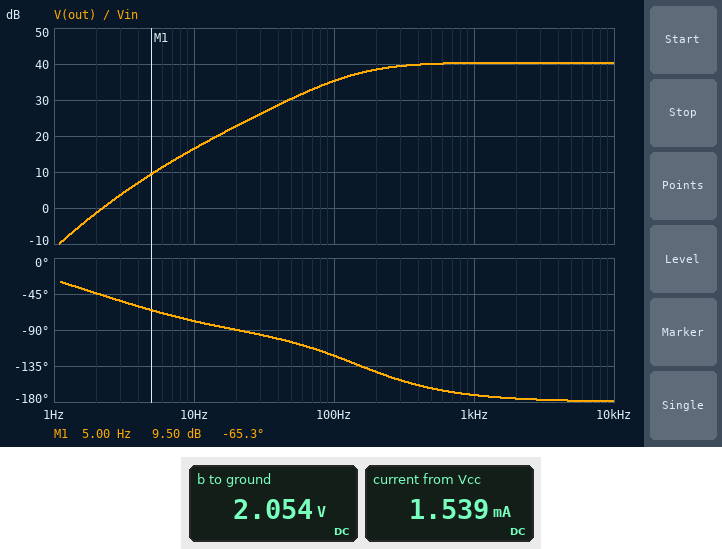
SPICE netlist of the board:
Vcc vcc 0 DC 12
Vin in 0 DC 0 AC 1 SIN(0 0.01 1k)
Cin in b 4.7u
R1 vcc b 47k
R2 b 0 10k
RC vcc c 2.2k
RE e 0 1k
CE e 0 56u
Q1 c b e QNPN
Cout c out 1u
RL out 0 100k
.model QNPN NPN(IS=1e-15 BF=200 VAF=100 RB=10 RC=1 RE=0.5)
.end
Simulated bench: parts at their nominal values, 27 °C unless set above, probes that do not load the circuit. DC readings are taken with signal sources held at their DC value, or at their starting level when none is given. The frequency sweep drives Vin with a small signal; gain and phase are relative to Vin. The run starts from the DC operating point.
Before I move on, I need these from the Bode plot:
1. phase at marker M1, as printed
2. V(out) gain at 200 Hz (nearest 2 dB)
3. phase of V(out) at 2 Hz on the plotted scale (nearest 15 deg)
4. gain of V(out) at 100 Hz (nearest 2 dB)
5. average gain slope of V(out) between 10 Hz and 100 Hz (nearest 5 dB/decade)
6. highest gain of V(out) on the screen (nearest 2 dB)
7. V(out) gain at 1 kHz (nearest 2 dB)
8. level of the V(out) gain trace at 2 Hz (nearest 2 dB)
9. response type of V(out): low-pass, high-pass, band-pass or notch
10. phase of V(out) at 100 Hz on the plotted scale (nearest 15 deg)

-65.3 deg
38 dB
-45 deg
36 dB
20 dB/decade
40 dB
40 dB
-2 dB
high-pass
-120 deg
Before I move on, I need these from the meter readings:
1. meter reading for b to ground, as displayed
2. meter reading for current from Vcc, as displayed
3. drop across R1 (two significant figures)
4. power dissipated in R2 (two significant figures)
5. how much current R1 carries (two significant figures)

2.054 V
1.539 mA
9.9 V
420 µW
210 µA
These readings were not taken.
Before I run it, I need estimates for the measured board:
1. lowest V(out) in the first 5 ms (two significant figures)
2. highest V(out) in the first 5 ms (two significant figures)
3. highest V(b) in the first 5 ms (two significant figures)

-1.1 V
960 mV
2.1 V
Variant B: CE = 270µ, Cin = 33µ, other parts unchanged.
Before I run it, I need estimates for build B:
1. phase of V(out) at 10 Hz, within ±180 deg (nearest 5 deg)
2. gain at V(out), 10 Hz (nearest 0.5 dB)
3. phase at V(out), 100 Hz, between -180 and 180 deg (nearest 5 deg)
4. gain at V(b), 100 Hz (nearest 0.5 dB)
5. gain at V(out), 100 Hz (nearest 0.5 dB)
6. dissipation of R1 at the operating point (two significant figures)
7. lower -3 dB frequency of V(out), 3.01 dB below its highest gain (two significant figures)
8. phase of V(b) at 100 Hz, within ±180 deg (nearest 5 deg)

-100 deg
30.0 dB
-160 deg
0 dB
40.0 dB
2.1 mW
31 Hz
0 deg
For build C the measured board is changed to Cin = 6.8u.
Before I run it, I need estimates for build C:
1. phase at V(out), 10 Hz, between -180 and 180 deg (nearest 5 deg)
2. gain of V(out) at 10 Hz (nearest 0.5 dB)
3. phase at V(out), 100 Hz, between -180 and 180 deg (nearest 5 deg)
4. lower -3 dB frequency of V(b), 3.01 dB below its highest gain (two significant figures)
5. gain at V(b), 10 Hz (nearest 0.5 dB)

-85 deg
17.0 dB
-125 deg
3.1 Hz
-0.5 dB
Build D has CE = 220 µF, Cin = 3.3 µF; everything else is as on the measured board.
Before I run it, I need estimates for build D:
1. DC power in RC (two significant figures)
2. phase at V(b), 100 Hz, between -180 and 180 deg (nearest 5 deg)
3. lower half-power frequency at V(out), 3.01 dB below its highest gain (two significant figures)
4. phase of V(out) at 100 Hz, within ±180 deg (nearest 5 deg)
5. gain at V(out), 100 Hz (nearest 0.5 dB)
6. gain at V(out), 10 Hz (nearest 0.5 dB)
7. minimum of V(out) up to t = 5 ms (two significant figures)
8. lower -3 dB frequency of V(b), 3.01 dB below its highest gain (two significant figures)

3.9 mW
10 deg
49 Hz
-150 deg
39.5 dB
25.5 dB
-1.2 V
12 Hz
